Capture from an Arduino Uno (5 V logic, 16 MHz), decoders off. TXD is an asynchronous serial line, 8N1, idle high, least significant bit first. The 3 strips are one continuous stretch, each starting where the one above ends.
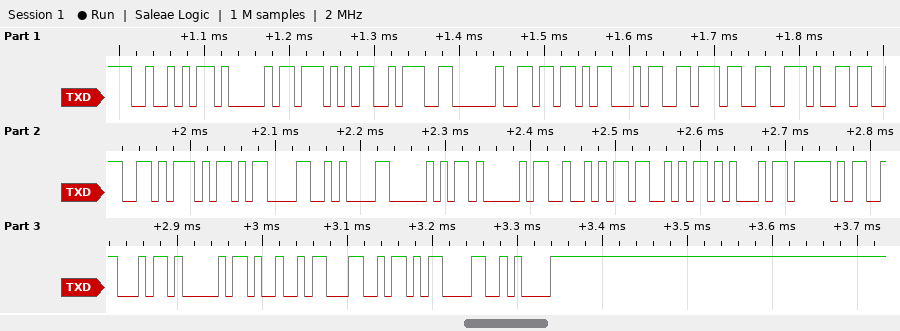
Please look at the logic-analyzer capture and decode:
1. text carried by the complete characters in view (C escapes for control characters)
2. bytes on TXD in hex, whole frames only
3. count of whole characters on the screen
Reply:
"RAW: [47.3]\r\nPARSE_FAIL\r\n"
52 41 57 3A 20 5B 34 37 2E 33 5D 0D 0A 50 41 52 53 45 5F 46 41 49 4C 0D 0A
25
